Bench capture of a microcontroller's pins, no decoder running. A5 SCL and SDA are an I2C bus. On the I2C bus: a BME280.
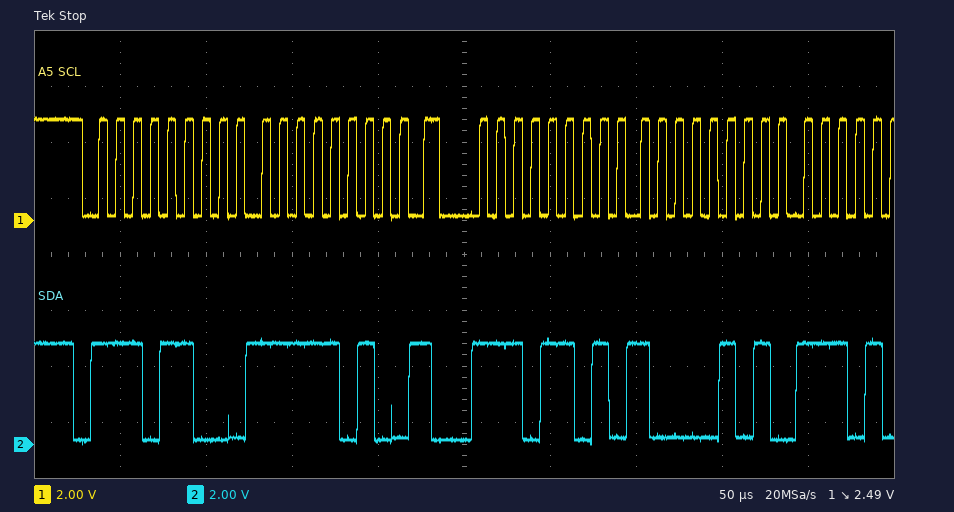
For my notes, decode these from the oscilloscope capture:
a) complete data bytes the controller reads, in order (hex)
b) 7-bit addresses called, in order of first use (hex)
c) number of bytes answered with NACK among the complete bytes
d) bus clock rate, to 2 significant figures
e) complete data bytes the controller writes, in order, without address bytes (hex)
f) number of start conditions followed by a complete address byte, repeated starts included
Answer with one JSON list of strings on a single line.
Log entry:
["85", "0x76", "0", "100 kHz", "FA", "2"]
